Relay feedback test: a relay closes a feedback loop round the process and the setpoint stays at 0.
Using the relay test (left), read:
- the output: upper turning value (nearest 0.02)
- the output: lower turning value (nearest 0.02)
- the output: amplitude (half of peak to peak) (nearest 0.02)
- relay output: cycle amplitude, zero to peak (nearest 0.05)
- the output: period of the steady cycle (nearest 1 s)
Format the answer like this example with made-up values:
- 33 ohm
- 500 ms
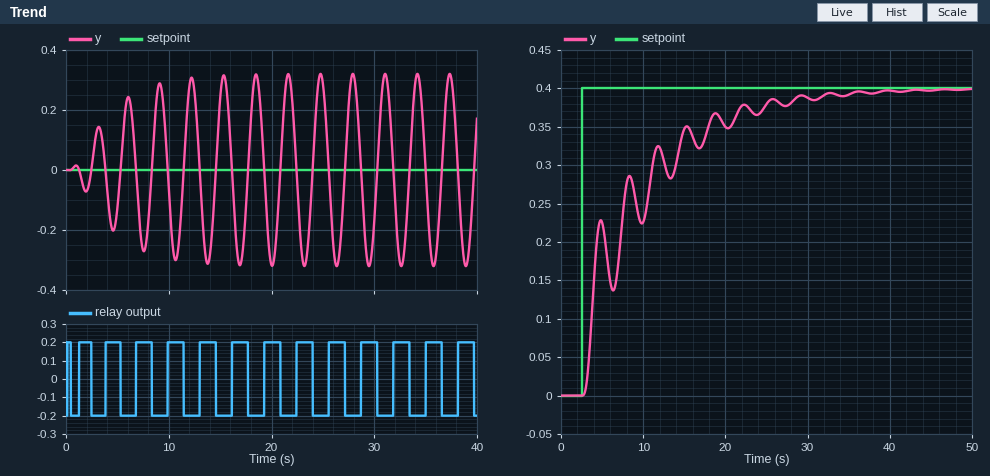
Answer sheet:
- 0.32
- -0.32
- 0.32
- 0.20
- 3 s
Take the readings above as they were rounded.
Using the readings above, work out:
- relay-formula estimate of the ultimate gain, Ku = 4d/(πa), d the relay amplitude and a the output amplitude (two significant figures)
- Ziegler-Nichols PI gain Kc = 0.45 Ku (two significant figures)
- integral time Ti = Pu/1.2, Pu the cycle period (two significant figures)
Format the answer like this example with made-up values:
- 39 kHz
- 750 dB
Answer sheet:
- 0.80
- 0.36
- 2.5 s
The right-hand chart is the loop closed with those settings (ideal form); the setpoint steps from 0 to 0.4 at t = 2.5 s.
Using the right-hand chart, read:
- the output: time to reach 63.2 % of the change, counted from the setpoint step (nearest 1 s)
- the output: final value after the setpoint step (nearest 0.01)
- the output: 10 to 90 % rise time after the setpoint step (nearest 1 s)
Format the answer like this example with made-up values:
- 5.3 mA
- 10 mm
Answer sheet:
- 5 s
- 0.40
- 15 s
